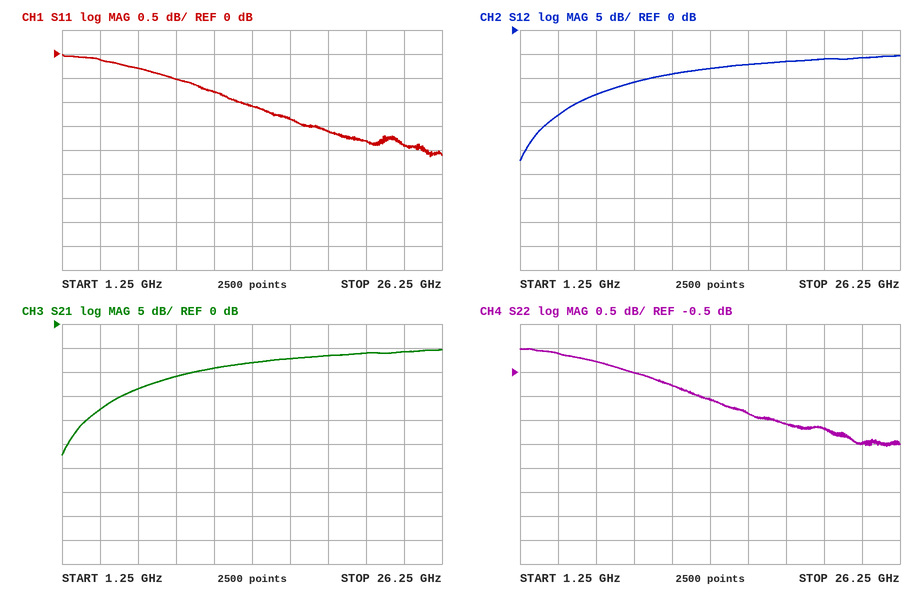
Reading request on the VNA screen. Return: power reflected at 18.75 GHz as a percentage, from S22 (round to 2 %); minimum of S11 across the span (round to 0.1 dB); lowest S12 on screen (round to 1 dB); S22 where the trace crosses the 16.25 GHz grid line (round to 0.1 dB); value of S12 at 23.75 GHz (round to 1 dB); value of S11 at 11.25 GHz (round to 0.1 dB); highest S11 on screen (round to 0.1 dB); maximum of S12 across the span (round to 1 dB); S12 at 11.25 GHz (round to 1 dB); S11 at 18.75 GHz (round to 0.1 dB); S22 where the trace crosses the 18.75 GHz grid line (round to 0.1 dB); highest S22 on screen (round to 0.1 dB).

70 %
-2.1 dB
-27 dB
-1.4 dB
-6 dB
-0.8 dB
0.0 dB
-5 dB
-9 dB
-1.6 dB
-1.6 dB
0.0 dB
